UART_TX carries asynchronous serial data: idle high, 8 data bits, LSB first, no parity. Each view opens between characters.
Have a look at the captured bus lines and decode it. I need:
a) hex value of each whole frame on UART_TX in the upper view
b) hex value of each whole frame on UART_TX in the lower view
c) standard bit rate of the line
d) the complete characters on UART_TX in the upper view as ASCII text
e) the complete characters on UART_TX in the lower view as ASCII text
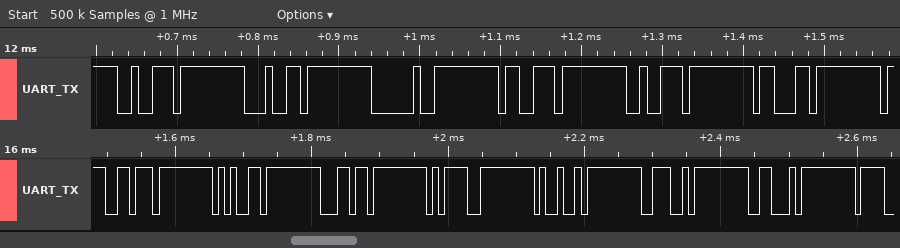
72, 64, 20, 73, 72, 63
76, 65, 6C, 3D, 49, 4E, 46
115200 baud
"rd src"
"vel=INF"
